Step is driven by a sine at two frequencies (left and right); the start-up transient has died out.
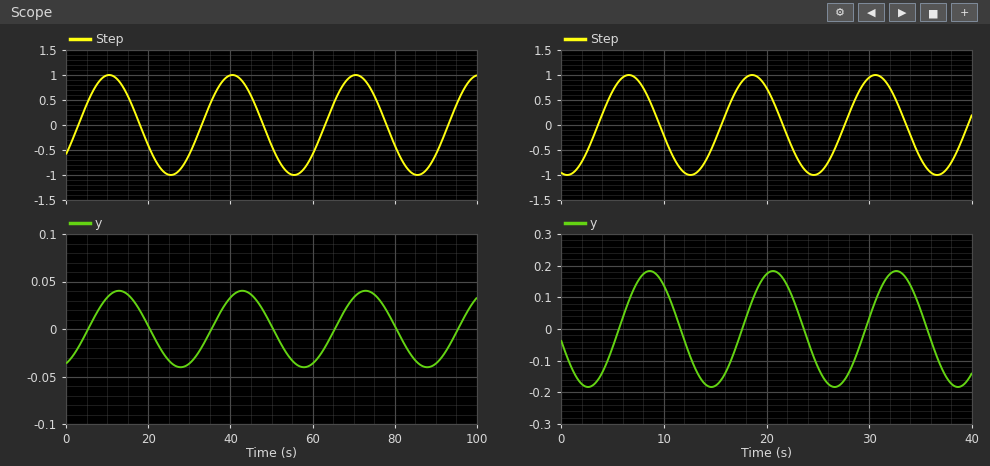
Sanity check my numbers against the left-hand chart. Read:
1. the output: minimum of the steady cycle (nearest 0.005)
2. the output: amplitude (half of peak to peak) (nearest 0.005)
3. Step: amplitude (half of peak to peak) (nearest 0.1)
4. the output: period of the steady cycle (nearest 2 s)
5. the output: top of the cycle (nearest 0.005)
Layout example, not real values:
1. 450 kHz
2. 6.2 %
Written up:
1. -0.040
2. 0.040
3. 1.0
4. 30 s
5. 0.040
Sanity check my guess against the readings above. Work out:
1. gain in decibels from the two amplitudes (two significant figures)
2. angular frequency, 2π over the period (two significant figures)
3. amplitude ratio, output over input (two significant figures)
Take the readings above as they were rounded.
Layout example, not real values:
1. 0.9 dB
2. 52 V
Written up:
1. -28 dB
2. 0.21 rad/s
3. 0.040
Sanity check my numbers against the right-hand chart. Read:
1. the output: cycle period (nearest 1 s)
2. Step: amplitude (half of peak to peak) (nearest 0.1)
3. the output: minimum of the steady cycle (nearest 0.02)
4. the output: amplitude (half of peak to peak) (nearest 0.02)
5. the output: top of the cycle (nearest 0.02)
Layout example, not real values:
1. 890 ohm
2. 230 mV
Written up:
1. 12 s
2. 1.0
3. -0.18
4. 0.18
5. 0.18
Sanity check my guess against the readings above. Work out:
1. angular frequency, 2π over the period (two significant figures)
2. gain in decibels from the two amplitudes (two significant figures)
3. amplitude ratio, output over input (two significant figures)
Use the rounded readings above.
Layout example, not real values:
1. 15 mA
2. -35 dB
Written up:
1. 0.52 rad/s
2. -15 dB
3. 0.18
